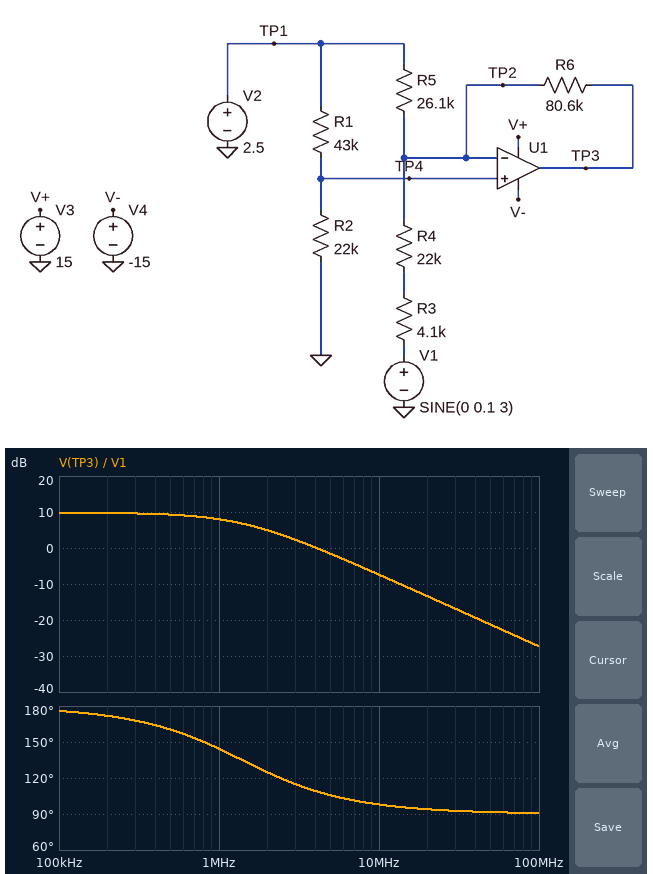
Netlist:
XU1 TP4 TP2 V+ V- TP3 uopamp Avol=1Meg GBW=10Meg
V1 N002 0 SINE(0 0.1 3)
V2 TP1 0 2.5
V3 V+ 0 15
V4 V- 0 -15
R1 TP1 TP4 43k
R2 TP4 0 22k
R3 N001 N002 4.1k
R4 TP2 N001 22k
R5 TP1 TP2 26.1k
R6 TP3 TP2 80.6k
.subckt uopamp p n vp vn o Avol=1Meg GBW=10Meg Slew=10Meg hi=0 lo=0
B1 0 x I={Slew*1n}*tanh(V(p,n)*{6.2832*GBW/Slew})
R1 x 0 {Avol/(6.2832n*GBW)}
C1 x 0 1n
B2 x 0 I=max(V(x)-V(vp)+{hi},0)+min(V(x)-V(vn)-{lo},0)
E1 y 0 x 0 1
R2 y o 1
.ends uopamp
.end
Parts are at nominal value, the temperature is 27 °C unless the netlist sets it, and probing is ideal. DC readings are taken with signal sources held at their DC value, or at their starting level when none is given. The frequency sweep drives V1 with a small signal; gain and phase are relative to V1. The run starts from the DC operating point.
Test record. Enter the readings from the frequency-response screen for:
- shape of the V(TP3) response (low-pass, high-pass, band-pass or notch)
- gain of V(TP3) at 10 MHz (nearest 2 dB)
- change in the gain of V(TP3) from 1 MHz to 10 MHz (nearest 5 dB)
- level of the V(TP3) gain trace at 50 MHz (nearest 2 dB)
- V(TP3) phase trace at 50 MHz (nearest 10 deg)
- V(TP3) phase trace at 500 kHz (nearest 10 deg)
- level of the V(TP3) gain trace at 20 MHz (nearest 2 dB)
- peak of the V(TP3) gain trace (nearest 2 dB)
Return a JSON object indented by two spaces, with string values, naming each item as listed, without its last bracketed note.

{
  "shape of the V(TP3) response": "low-pass",
  "gain of V(TP3) at 10 MHz": "-8 dB",
  "change in the gain of V(TP3) from 1 MHz to 10 MHz": "-15 dB",
  "level of the V(TP3) gain trace at 50 MHz": "-22 dB",
  "V(TP3) phase trace at 50 MHz": "90 deg",
  "V(TP3) phase trace at 500 kHz": "160 deg",
  "level of the V(TP3) gain trace at 20 MHz": "-14 dB",
  "peak of the V(TP3) gain trace": "10 dB"
}
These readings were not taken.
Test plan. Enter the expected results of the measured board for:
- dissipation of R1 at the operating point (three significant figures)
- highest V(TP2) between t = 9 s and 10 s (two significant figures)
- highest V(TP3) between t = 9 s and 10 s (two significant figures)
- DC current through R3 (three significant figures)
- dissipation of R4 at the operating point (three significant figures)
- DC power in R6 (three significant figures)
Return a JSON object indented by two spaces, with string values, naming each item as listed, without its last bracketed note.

{
  "dissipation of R1 at the operating point": "63.6 µW",
  "highest V(TP2) between t = 9 s and 10 s": "850 mV",
  "highest V(TP3) between t = 9 s and 10 s": "-1.3 V",
  "DC current through R3": "32.4 µA",
  "dissipation of R4 at the operating point": "23.1 µW",
  "DC power in R6": "77.2 µW"
}
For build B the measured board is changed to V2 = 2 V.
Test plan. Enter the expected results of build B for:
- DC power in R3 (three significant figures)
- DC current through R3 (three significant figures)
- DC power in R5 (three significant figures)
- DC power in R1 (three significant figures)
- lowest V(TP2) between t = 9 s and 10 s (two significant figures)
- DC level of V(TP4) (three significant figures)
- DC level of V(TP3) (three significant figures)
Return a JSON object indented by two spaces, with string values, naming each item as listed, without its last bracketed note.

{
  "DC power in R3": "2.76 µW",
  "DC current through R3": "25.9 µA",
  "DC power in R5": "67.1 µW",
  "DC power in R1": "40.7 µW",
  "lowest V(TP2) between t = 9 s and 10 s": "680 mV",
  "DC level of V(TP4)": "677 mV",
  "DC level of V(TP3)": "-1.32 V"
}
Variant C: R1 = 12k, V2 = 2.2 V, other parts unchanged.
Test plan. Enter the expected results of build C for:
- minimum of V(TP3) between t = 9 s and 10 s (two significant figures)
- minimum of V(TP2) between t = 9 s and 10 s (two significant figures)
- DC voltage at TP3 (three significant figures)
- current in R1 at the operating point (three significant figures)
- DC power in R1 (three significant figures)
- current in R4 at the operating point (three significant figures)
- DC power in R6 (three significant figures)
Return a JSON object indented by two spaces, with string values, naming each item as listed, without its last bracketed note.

{
  "minimum of V(TP3) between t = 9 s and 10 s": "3.1 V",
  "minimum of V(TP2) between t = 9 s and 10 s": "1.4 V",
  "DC voltage at TP3": "3.42 V",
  "current in R1 at the operating point": "64.7 µA",
  "DC power in R1": "50.2 µW",
  "current in R4 at the operating point": "54.5 µA",
  "DC power in R6": "49.5 µW"
}
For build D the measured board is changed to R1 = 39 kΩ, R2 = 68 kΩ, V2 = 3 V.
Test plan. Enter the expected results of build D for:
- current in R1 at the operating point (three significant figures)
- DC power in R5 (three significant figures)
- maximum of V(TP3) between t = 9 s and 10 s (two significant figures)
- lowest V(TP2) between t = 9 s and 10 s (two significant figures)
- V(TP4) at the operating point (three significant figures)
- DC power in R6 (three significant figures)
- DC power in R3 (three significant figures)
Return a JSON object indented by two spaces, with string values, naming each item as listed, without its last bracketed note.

{
  "current in R1 at the operating point": "28.0 µA",
  "DC power in R5": "45.8 µW",
  "maximum of V(TP3) between t = 9 s and 10 s": "4.7 V",
  "lowest V(TP2) between t = 9 s and 10 s": "1.9 V",
  "V(TP4) at the operating point": "1.91 V",
  "DC power in R6": "78.2 µW",
  "DC power in R3": "21.9 µW"
}
